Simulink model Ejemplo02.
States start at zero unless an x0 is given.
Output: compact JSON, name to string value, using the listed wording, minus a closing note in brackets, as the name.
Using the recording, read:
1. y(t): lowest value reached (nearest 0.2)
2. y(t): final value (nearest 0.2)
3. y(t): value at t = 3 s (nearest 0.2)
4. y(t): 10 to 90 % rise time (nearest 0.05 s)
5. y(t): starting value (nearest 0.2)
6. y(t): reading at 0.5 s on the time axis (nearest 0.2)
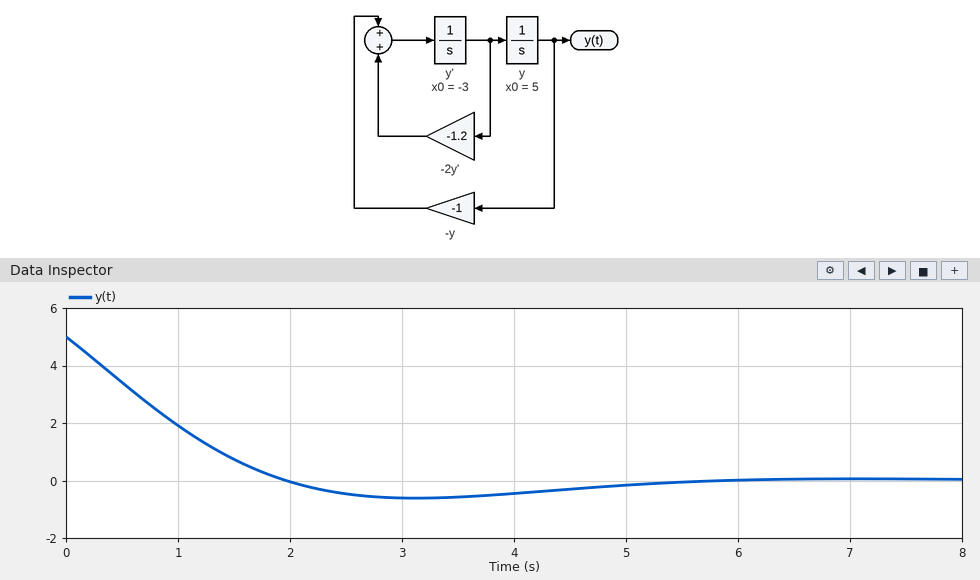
{"y(t): lowest value reached": "-0.6", "y(t): final value": "0.0", "y(t): value at t = 3 s": "-0.6", "y(t): 10 to 90 % rise time": "1.45 s", "y(t): starting value": "5.0", "y(t): reading at 0.5 s on the time axis": "3.4"}
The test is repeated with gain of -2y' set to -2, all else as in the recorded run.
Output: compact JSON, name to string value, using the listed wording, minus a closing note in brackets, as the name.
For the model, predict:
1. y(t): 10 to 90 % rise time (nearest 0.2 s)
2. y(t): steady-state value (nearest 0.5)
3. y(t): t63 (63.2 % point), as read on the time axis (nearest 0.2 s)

{"y(t): 10 to 90 % rise time": "3.0 s", "y(t): steady-state value": "0.0", "y(t): t63 (63.2 % point), as read on the time axis": "1.4 s"}
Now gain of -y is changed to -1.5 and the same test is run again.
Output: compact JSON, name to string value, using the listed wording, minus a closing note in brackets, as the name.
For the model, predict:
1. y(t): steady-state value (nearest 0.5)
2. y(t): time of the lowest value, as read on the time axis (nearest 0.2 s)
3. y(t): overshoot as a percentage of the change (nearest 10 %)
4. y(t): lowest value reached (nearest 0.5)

{"y(t): steady-state value": "0.0", "y(t): time of the lowest value, as read on the time axis": "2.4 s", "y(t): overshoot as a percentage of the change": "20 %", "y(t): lowest value reached": "-1.0"}
